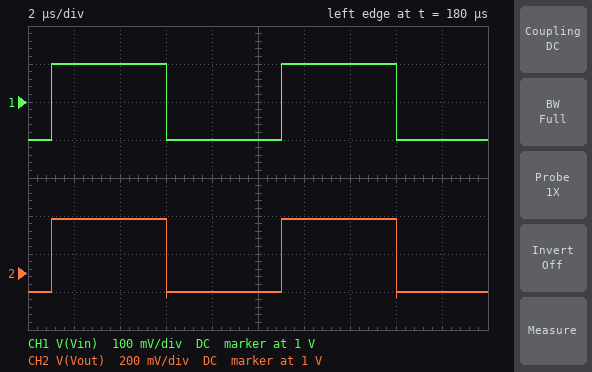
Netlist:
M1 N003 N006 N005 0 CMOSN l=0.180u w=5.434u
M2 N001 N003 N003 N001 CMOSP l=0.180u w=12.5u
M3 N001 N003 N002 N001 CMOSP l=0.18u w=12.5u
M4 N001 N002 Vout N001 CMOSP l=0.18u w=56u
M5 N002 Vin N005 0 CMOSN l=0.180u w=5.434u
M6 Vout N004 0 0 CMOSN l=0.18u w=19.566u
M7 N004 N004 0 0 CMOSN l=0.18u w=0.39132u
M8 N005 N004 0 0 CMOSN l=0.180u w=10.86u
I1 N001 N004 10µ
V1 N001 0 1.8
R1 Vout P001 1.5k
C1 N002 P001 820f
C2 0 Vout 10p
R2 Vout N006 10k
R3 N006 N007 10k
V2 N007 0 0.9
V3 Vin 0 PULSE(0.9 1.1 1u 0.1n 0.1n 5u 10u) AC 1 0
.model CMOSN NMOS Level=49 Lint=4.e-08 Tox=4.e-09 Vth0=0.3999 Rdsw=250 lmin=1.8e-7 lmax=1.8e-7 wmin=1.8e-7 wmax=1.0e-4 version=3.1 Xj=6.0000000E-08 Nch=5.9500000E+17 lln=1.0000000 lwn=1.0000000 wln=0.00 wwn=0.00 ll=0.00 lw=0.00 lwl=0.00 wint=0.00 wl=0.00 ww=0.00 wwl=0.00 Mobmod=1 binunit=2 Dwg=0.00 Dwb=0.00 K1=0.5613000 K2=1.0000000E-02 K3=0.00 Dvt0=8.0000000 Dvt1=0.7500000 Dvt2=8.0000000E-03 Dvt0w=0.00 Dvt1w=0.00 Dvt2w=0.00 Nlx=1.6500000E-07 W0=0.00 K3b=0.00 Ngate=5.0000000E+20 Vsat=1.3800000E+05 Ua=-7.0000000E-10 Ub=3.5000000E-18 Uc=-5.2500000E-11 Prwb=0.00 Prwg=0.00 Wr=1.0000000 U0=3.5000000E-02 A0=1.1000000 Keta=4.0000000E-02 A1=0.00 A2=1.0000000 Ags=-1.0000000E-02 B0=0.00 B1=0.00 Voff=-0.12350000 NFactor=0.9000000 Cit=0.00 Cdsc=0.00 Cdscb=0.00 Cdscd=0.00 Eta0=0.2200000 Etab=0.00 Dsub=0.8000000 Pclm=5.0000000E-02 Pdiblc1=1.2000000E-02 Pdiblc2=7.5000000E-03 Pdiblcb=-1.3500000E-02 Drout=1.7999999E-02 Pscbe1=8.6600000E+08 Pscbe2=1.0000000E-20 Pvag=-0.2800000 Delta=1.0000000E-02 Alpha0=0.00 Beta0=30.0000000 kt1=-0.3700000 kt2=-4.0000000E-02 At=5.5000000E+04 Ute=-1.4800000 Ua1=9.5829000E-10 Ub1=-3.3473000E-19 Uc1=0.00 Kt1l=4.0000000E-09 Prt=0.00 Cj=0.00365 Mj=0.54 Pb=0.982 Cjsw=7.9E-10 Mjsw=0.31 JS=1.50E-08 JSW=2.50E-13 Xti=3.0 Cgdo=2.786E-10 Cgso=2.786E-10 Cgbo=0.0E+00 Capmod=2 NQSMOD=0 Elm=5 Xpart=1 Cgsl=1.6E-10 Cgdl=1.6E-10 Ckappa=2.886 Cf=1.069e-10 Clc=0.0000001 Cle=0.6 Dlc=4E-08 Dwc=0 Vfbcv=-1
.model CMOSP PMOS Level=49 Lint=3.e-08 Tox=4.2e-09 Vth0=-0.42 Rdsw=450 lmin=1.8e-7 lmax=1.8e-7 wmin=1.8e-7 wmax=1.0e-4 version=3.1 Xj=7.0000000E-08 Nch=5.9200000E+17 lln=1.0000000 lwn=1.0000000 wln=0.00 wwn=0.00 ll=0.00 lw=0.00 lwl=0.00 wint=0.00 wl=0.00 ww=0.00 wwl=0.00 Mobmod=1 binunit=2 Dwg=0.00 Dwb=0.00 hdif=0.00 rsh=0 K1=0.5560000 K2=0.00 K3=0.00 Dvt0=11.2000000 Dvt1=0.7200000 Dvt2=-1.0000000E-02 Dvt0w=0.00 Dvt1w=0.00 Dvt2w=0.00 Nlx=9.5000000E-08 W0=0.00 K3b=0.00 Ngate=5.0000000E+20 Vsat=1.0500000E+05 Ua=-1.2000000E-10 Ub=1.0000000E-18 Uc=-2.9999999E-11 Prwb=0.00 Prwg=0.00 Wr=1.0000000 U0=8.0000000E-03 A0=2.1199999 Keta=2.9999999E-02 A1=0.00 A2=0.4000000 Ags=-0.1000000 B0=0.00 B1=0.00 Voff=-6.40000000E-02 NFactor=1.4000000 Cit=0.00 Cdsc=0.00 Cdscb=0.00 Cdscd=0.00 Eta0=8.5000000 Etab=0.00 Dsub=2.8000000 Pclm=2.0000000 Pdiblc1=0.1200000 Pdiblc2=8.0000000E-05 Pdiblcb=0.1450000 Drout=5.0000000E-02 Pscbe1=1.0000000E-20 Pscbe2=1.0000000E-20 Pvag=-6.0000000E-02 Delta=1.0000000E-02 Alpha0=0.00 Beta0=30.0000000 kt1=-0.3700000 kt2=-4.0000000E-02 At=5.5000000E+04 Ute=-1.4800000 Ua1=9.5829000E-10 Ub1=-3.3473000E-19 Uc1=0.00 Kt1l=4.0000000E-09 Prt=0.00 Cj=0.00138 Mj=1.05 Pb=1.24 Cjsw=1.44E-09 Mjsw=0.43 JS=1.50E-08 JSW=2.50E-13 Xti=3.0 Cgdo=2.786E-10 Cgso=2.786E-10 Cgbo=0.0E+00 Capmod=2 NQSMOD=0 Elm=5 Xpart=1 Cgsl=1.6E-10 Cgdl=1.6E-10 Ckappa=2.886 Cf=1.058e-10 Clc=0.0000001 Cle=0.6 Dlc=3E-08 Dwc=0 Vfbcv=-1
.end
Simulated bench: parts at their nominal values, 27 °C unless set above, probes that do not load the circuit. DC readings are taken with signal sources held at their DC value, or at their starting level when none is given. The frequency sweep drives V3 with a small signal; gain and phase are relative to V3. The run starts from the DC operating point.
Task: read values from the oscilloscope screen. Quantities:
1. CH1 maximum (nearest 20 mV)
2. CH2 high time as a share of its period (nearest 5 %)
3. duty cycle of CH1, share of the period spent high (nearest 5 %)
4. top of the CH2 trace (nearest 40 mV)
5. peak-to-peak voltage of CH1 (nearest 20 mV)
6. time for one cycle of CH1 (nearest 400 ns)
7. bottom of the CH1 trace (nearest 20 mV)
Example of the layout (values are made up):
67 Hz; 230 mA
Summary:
1.10 V; 50 %; 50 %; 1.28 V; 200 mV; 10.0 µs; 900 mV
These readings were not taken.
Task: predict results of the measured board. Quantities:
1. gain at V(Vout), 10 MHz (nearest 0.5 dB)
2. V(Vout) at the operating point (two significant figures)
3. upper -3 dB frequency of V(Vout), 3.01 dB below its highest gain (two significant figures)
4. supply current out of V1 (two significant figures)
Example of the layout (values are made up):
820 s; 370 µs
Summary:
5.5 dB; 900 mV; 91 MHz; 920 µA
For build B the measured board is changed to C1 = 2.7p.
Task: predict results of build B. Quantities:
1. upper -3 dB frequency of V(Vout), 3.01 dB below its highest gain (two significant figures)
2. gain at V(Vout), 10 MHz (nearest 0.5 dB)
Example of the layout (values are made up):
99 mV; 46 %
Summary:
26 MHz; 5.0 dB
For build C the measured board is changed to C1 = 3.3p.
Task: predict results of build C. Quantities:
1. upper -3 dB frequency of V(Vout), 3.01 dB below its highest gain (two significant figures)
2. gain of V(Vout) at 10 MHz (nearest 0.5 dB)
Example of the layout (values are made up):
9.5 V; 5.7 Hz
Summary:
21 MHz; 4.5 dB
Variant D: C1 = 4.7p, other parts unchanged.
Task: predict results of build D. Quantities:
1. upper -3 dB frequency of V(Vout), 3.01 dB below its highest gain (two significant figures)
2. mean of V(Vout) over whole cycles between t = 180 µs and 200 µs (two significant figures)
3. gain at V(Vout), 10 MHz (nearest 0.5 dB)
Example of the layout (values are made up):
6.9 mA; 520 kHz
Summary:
14 MHz; 1.1 V; 4.0 dB
